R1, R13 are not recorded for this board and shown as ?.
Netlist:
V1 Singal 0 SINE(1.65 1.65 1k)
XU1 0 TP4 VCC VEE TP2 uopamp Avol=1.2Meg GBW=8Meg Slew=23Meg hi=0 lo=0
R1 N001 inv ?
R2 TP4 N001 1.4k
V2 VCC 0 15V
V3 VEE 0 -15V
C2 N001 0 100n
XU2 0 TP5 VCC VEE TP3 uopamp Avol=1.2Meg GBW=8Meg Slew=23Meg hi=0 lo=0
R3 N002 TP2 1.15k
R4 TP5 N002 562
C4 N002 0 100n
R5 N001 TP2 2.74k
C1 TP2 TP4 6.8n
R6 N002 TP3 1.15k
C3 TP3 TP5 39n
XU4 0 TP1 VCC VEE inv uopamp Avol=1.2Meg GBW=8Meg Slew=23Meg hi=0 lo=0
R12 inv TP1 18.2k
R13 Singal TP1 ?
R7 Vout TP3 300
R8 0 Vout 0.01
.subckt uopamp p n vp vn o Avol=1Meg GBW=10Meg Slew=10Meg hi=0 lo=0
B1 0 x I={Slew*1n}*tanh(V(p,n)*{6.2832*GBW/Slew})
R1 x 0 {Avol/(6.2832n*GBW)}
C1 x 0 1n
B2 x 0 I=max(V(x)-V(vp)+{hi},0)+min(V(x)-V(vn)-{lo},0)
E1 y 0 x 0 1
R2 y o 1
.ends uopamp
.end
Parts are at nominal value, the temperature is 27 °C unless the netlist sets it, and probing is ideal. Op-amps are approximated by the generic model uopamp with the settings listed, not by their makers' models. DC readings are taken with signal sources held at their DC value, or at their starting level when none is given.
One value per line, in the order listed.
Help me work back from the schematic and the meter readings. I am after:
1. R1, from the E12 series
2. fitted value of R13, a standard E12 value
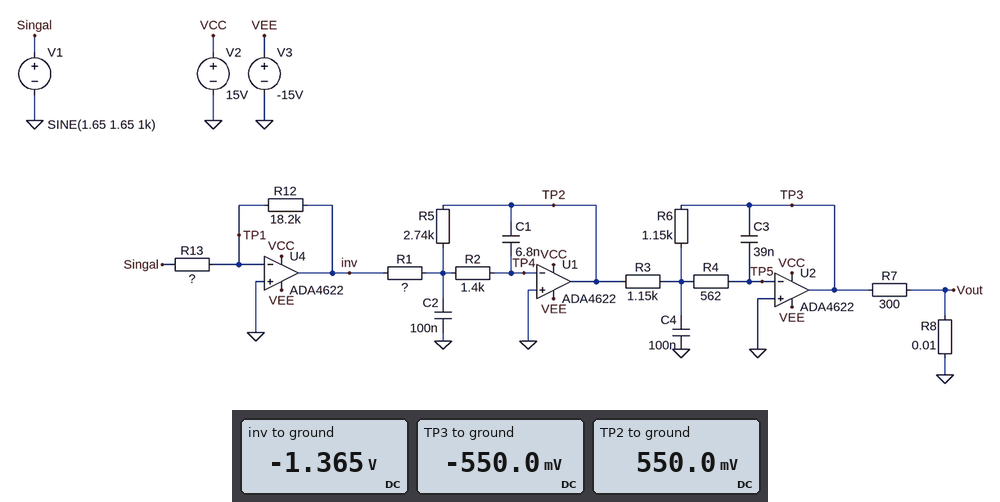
6.8 kΩ
22 kΩ
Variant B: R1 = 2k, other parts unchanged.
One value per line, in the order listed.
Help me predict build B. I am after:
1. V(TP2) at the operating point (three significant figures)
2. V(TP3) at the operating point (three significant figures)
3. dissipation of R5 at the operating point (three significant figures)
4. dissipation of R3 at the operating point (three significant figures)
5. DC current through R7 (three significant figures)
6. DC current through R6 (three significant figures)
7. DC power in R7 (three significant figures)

1.87 V
-1.87 V
1.28 mW
3.04 mW
6.23 mA
1.63 mA
11.7 mW
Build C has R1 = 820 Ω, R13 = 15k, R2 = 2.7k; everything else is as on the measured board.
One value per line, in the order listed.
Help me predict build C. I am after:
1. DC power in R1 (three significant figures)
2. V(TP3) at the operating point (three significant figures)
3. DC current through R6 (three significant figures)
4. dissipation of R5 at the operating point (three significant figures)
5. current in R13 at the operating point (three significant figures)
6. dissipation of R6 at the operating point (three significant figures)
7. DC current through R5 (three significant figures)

4.89 mW
-6.69 V
5.82 mA
16.3 mW
110 µA
38.9 mW
2.44 mA
